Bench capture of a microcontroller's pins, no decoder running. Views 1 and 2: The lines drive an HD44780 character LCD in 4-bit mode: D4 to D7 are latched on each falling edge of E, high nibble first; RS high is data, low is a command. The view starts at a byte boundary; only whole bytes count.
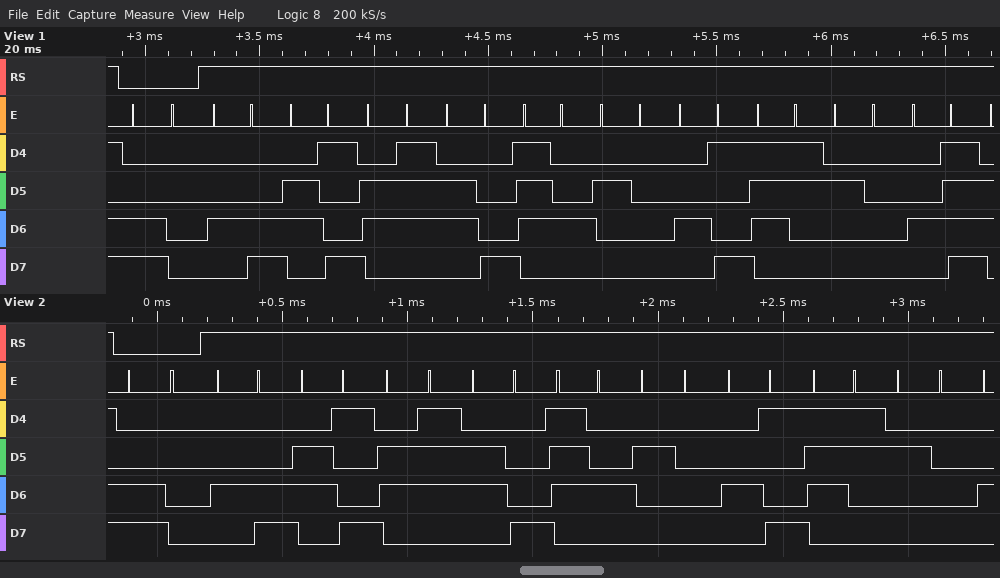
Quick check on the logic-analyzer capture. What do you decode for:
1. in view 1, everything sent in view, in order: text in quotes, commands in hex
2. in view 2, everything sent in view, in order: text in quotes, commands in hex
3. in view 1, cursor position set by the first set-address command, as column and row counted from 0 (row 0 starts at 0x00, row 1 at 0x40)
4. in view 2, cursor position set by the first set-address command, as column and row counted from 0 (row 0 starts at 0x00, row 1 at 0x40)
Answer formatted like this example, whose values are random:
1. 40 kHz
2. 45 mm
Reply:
1. 0xC0 "Light Is O"
2. 0xC0 "Light Is "
3. column 0, row 1
4. column 0, row 1
